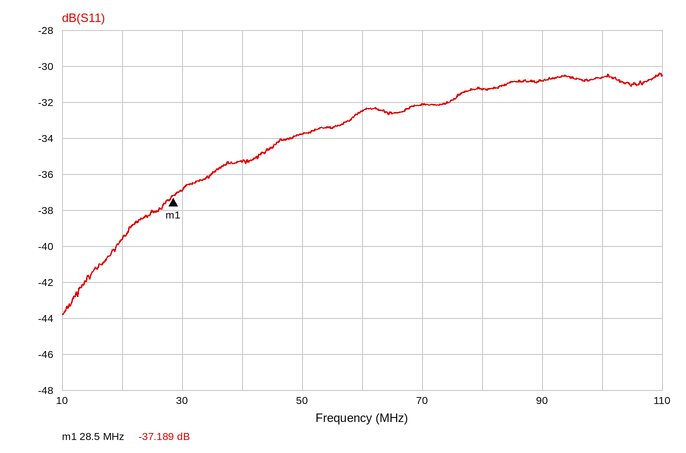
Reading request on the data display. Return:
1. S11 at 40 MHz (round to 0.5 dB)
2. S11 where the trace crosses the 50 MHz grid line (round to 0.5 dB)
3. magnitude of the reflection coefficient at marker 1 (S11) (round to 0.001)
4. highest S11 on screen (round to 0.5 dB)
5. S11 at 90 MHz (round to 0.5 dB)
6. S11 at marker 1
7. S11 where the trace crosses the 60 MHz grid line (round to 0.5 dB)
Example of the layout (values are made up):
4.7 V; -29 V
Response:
-35.5 dB; -34.0 dB; 0.014; -30.5 dB; -31.0 dB; -37.189 dB; -32.5 dB
